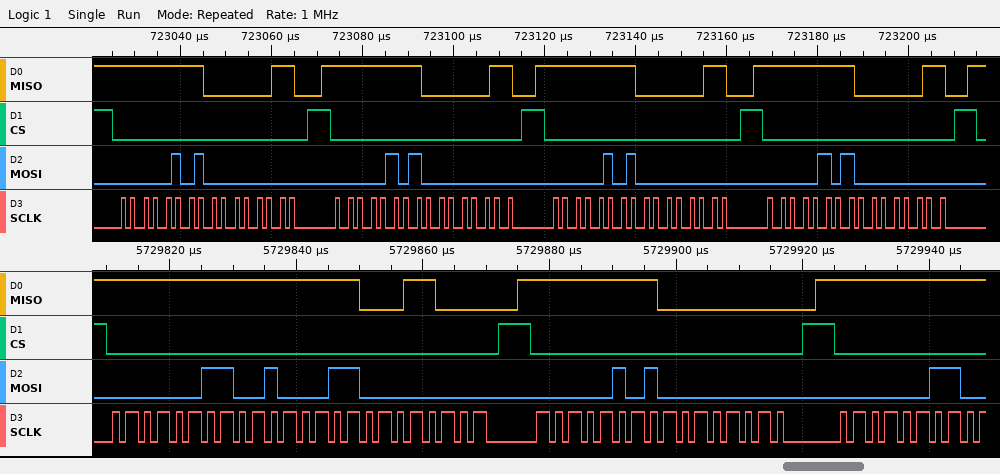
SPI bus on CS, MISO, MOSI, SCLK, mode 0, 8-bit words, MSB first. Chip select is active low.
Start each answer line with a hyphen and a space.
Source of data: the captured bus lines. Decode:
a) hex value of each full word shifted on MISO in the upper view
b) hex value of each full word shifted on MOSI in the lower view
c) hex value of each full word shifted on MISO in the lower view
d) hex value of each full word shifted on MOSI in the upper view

- FF, 03, FF, 03, FF, 03, FF, 03
- 03, 23, 00, 05, 00, 03
- FF, FF, 18, FF, 00, FF
- 05, 00, 05, 00, 05, 00, 05, 00
